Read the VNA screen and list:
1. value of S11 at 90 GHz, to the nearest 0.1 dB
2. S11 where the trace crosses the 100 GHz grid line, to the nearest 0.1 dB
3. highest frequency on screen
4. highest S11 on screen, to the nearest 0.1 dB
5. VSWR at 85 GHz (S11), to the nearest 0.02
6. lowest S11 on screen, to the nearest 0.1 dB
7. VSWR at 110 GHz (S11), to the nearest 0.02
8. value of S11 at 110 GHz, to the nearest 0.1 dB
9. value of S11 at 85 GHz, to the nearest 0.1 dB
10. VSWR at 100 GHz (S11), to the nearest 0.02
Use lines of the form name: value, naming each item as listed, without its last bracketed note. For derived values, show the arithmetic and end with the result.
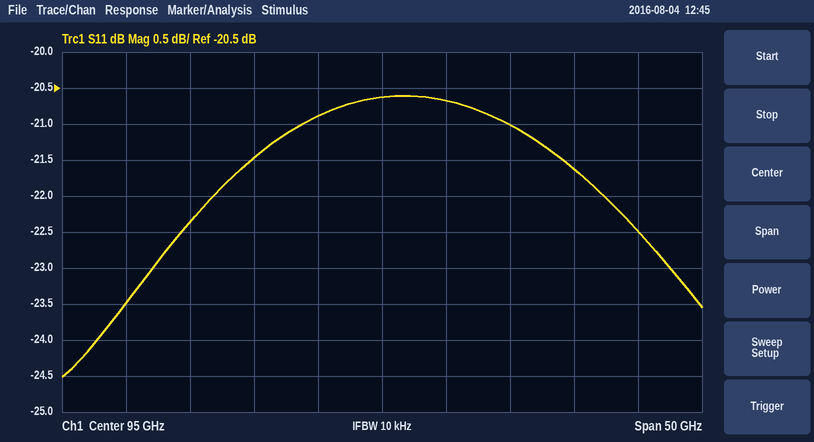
value of S11 at 90 GHz, to the nearest 0.1 dB: -20.9 dB
S11 where the trace crosses the 100 GHz grid line, to the nearest 0.1 dB: -20.7 dB
highest frequency on screen: 120 GHz
highest S11 on screen, to the nearest 0.1 dB: -20.6 dB
VSWR at 85 GHz (S11), to the nearest 0.02: |Γ| = 10^(-21.5/20) = 0.0841; VSWR = (1 + 0.0841)/(1 − 0.0841) ≈ 1.18
lowest S11 on screen, to the nearest 0.1 dB: -24.5 dB
VSWR at 110 GHz (S11), to the nearest 0.02: |Γ| = 10^(-21.6/20) = 0.0832; VSWR = (1 + 0.0832)/(1 − 0.0832) ≈ 1.18
value of S11 at 110 GHz, to the nearest 0.1 dB: -21.6 dB
value of S11 at 85 GHz, to the nearest 0.1 dB: -21.5 dB
VSWR at 100 GHz (S11), to the nearest 0.02: |Γ| = 10^(-20.7/20) = 0.0923; VSWR = (1 + 0.0923)/(1 − 0.0923) ≈ 1.20
